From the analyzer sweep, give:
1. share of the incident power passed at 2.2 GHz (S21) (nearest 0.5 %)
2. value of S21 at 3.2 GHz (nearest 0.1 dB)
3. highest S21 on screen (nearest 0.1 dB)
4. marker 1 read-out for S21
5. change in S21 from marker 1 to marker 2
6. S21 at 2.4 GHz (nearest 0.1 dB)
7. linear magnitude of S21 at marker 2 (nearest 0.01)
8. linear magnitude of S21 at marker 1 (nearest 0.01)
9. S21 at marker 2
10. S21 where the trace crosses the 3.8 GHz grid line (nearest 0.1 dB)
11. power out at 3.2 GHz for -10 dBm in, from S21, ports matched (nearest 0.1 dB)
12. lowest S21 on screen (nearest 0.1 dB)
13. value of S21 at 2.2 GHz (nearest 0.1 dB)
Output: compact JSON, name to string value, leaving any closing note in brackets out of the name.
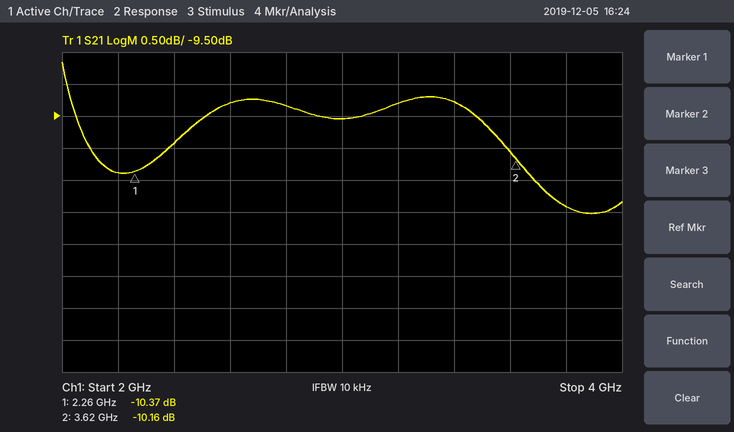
{"share of the incident power passed at 2.2 GHz (S21)": "9.0 %", "value of S21 at 3.2 GHz": "-9.3 dB", "highest S21 on screen": "-8.7 dB", "marker 1 read-out for S21": "-10.37 dB", "change in S21 from marker 1 to marker 2": "0.21 dB", "S21 at 2.4 GHz": "-9.9 dB", "linear magnitude of S21 at marker 2": "0.31", "linear magnitude of S21 at marker 1": "0.30", "S21 at marker 2": "-10.16 dB", "S21 where the trace crosses the 3.8 GHz grid line": "-10.9 dB", "power out at 3.2 GHz for -10 dBm in, from S21, ports matched": "-19.3 dBm", "lowest S21 on screen": "-11.0 dB", "value of S21 at 2.2 GHz": "-10.4 dB"}
